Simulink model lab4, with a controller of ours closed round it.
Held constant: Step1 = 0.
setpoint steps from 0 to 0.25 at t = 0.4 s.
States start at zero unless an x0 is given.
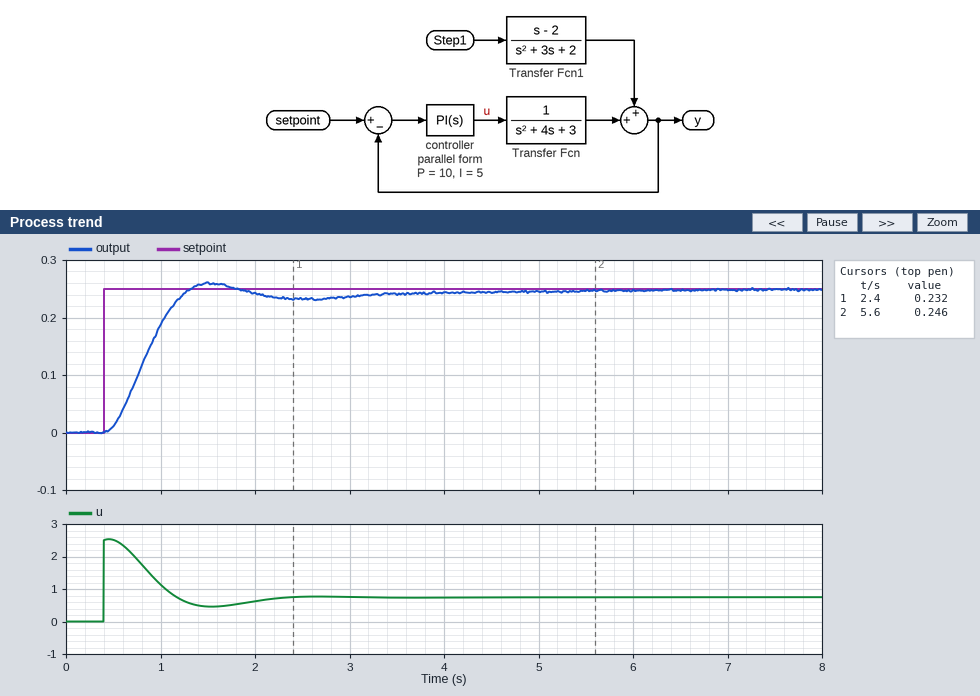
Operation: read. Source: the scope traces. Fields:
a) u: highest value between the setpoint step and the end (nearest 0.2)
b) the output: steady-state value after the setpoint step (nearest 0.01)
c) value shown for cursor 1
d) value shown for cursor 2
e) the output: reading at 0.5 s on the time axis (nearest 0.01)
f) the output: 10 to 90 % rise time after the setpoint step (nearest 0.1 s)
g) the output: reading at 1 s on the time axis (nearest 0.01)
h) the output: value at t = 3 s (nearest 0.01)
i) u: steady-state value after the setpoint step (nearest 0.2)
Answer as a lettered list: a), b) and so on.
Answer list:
a) 2.6
b) 0.25
c) 0.232
d) 0.246
e) 0.01
f) 0.6 s
g) 0.19
h) 0.24
i) 0.8
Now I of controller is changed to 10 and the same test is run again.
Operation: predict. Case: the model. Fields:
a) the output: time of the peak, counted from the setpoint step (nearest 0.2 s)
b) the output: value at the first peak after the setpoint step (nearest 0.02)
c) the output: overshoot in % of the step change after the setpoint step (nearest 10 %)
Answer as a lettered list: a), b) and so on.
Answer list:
a) 1.2 s
b) 0.30
c) 20 %
